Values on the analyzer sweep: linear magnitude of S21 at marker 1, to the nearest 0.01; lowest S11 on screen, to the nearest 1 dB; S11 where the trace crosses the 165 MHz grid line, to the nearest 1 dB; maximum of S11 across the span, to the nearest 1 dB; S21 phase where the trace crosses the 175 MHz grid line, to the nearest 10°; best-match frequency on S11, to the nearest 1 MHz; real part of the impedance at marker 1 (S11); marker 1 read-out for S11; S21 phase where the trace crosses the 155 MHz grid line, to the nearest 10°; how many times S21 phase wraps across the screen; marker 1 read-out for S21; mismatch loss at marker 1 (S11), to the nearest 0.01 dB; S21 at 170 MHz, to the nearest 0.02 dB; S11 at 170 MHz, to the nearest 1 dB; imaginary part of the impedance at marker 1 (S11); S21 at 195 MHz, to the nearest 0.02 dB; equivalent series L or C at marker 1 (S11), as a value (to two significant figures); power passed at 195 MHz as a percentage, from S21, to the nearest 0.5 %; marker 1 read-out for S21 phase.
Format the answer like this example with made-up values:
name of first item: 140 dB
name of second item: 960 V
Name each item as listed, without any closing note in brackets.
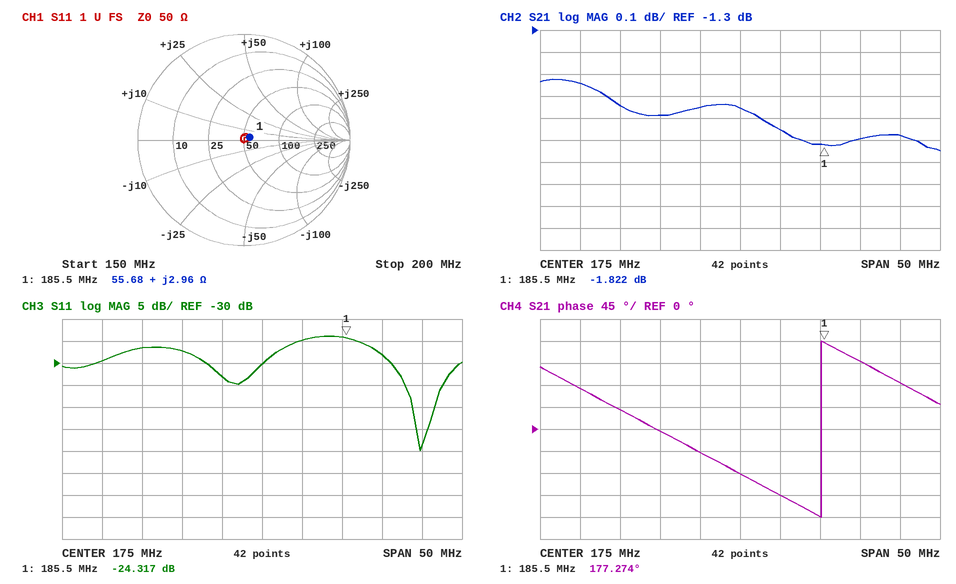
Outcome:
linear magnitude of S21 at marker 1, to the nearest 0.01: 0.81
lowest S11 on screen, to the nearest 1 dB: -50 dB
S11 where the trace crosses the 165 MHz grid line, to the nearest 1 dB: -27 dB
maximum of S11 across the span, to the nearest 1 dB: -24 dB
S21 phase where the trace crosses the 175 MHz grid line, to the nearest 10°: -90°
best-match frequency on S11, to the nearest 1 MHz: 195 MHz
real part of the impedance at marker 1: 55.68 Ω
marker 1 read-out for S11: -24.317 dB
S21 phase where the trace crosses the 155 MHz grid line, to the nearest 10°: 80°
how many times S21 phase wraps across the screen: 1
marker 1 read-out for S21: -1.822 dB
mismatch loss at marker 1 (S11), to the nearest 0.01 dB: 0.02 dB
S21 at 170 MHz, to the nearest 0.02 dB: -1.66 dB
S11 at 170 MHz, to the nearest 1 dB: -33 dB
imaginary part of the impedance at marker 1: +2.96 Ω
S21 at 195 MHz, to the nearest 0.02 dB: -1.78 dB
equivalent series L or C at marker 1 (S11), as a value: 2.5 nH
power passed at 195 MHz as a percentage, from S21, to the nearest 0.5 %: 66.5 %
marker 1 read-out for S21 phase: 177.274°
